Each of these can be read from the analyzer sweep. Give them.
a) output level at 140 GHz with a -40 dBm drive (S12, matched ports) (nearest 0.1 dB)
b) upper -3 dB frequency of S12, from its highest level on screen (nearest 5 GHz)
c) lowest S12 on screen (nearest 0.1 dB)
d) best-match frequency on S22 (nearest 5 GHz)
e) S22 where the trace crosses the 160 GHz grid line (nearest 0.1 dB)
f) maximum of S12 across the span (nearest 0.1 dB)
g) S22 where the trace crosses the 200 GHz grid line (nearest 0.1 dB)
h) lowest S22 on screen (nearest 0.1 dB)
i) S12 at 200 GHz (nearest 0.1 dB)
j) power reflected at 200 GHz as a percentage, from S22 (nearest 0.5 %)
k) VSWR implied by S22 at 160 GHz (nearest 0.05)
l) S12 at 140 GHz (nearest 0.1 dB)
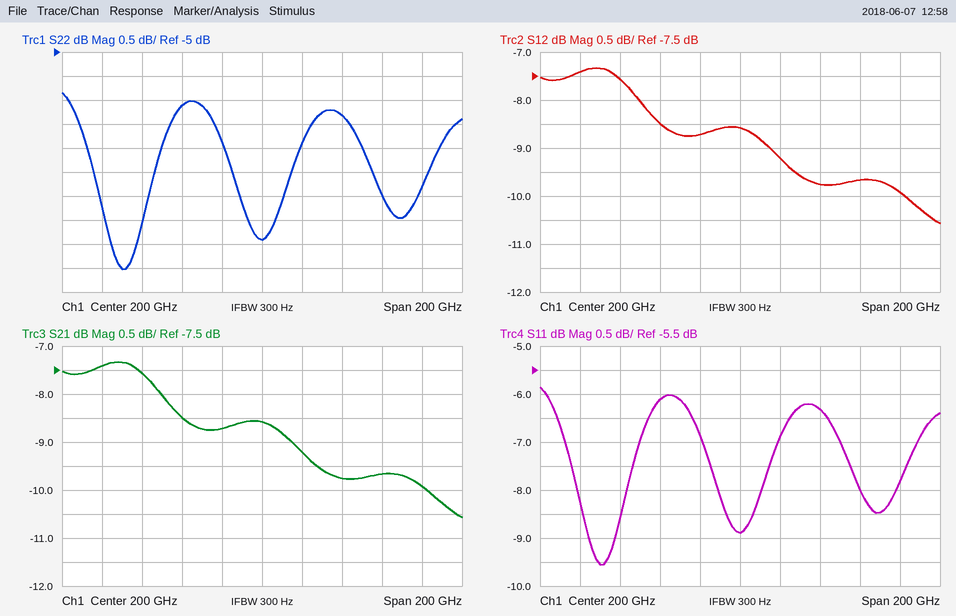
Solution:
-47.6 dBm
290 GHz
-10.6 dB
130 GHz
-6.1 dB
-7.3 dB
-8.9 dB
-9.5 dB
-8.6 dB
13.0 %
2.95
-7.6 dB
